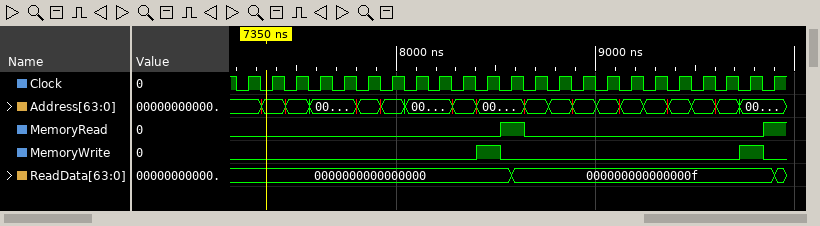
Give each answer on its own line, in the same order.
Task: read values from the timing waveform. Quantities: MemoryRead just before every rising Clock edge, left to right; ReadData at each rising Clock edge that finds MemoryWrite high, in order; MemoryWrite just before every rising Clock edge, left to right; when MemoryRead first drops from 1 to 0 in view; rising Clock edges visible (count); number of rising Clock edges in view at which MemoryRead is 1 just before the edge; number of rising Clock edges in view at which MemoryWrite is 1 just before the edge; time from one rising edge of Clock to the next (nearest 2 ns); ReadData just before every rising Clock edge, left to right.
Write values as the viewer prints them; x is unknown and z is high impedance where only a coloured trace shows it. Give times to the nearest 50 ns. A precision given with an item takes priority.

0 0 0 0 0 0 0 0 0 0 0 1 0 0 0 0 0 0 0 0 0 0 1
0000000000000000, 000000000000000f
0 0 0 0 0 0 0 0 0 0 1 0 0 0 0 0 0 0 0 0 0 1 0
8650 ns
23
2
2
120 ns
0000000000000000, 0000000000000000, 0000000000000000, 0000000000000000, 0000000000000000, 0000000000000000, 0000000000000000, 0000000000000000, 0000000000000000, 0000000000000000, 0000000000000000, 0000000000000000, 000000000000000f, 000000000000000f, 000000000000000f, 000000000000000f, 000000000000000f, 000000000000000f, 000000000000000f, 000000000000000f, 000000000000000f, 000000000000000f, 000000000000000f
